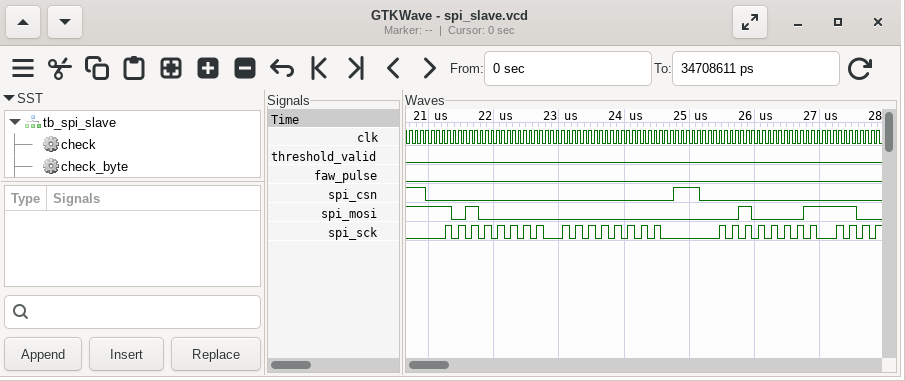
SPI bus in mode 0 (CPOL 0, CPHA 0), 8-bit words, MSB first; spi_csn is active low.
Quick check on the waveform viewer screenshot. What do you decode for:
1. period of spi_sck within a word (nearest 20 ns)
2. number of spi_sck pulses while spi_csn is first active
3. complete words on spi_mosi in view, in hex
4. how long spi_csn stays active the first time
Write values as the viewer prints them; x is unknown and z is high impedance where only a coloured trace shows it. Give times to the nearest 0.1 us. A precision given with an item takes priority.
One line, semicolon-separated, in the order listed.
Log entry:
200 ns; 16; A0, 00, 21; 3.8 us
